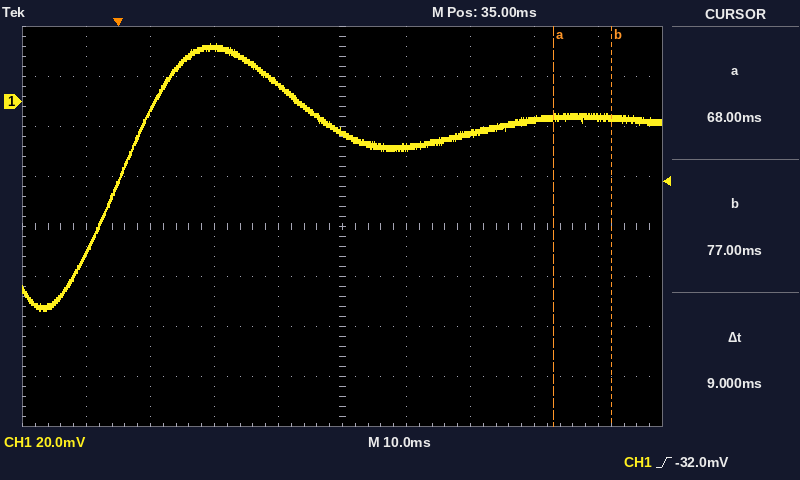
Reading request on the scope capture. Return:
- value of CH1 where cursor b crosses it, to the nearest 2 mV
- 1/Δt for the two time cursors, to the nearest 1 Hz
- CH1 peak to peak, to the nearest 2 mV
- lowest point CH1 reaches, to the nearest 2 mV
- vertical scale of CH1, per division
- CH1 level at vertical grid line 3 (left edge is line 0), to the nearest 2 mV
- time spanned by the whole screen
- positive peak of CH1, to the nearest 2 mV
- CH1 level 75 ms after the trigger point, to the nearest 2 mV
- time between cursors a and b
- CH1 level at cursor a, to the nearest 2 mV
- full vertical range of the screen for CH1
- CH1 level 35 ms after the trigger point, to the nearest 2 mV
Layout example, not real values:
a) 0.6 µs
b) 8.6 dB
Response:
a) -6 mV
b) 111 Hz
c) 108 mV
d) -84 mV
e) 20 mV
f) 22 mV
g) 100 ms
h) 24 mV
i) -6 mV
j) 9 ms
k) -6 mV
l) 160 mV
m) -12 mV
